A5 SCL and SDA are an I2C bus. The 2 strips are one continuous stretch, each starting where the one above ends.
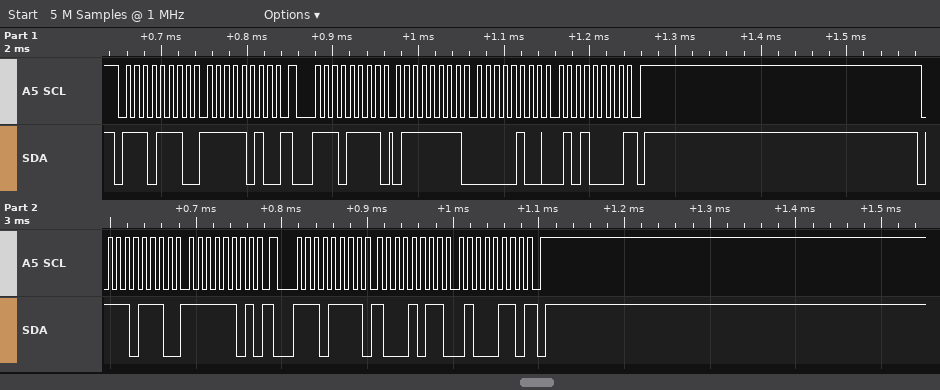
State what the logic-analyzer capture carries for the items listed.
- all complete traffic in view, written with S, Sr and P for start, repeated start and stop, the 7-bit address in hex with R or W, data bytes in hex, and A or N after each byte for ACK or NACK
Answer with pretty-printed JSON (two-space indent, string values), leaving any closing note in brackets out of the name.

{
  "all complete traffic in view, written with S, Sr and P for start, repeated start and stop, the 7-bit address in hex with R or W, data bytes in hex, and A or N after each byte for ACK or NACK": "S 77W A FA A Sr 77R A 7F A 04 A 50 N P S 77W A FD A Sr 77R A 8B A 46 N P"
}
